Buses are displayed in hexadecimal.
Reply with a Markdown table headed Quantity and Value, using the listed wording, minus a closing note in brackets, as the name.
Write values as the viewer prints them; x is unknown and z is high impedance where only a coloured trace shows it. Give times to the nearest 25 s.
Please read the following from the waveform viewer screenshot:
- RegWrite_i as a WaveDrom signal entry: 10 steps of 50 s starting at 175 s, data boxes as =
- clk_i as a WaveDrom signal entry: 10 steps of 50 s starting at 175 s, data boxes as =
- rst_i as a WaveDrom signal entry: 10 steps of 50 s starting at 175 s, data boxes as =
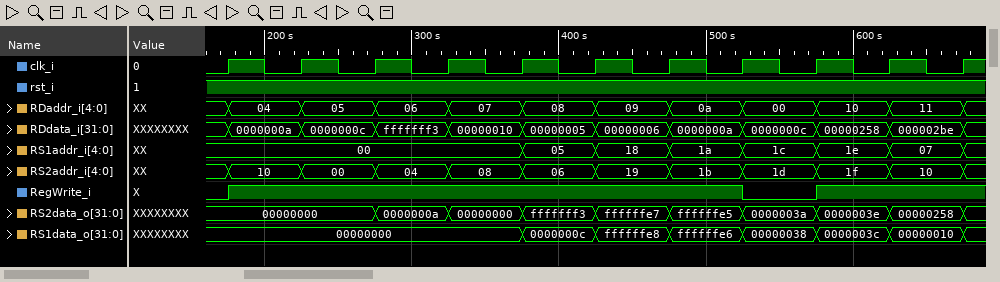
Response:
| Quantity | Value |
|---|---|
| RegWrite_i as a WaveDrom signal entry: 10 steps of 50 s starting at 175 s, data boxes as = | {name: 'RegWrite_i', wave: '1......01.'} |
| clk_i as a WaveDrom signal entry: 10 steps of 50 s starting at 175 s, data boxes as = | {name: 'clk_i', wave: 'p.........'} |
| rst_i as a WaveDrom signal entry: 10 steps of 50 s starting at 175 s, data boxes as = | {name: 'rst_i', wave: '1.........'} |
